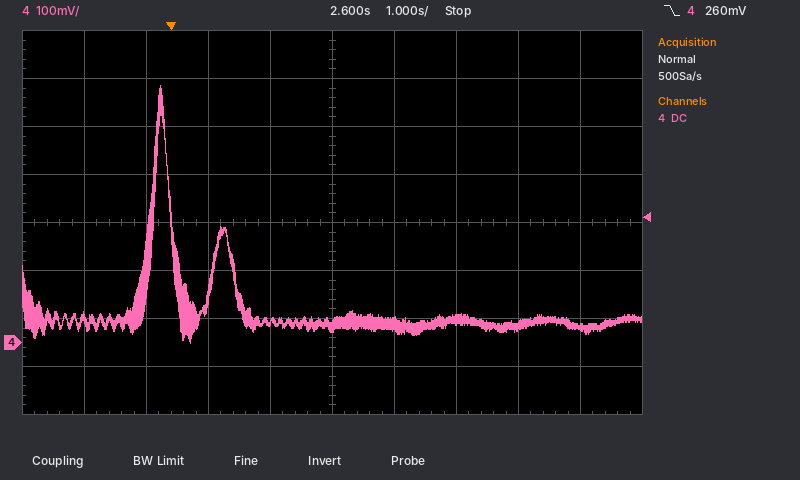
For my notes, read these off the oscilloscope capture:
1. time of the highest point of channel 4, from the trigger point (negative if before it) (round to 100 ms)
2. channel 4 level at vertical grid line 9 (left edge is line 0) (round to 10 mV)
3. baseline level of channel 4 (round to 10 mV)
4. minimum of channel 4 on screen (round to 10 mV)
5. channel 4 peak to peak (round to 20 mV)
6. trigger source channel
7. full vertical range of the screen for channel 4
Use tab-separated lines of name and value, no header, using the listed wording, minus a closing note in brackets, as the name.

time of the highest point of channel 4, from the trigger point (negative if before it)	-200 ms
channel 4 level at vertical grid line 9 (left edge is line 0)	30 mV
baseline level of channel 4	40 mV
minimum of channel 4 on screen	0 mV
channel 4 peak to peak	540 mV
trigger source channel	channel 4
full vertical range of the screen for channel 4	800 mV
